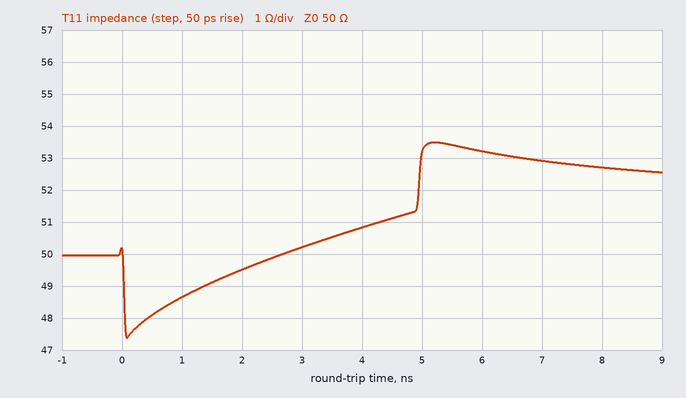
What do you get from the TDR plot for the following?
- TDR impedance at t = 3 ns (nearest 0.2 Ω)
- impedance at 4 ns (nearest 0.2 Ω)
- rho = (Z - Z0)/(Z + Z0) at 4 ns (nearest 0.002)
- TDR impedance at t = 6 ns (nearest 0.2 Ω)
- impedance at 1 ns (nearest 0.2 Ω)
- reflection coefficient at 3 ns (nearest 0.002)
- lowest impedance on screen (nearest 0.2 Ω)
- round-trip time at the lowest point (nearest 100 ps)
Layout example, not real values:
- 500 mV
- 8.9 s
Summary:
- 50.2 Ω
- 50.8 Ω
- +0.008
- 53.2 Ω
- 48.6 Ω
- +0.002
- 47.4 Ω
- 100 ps
